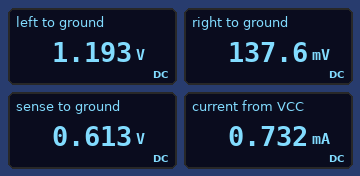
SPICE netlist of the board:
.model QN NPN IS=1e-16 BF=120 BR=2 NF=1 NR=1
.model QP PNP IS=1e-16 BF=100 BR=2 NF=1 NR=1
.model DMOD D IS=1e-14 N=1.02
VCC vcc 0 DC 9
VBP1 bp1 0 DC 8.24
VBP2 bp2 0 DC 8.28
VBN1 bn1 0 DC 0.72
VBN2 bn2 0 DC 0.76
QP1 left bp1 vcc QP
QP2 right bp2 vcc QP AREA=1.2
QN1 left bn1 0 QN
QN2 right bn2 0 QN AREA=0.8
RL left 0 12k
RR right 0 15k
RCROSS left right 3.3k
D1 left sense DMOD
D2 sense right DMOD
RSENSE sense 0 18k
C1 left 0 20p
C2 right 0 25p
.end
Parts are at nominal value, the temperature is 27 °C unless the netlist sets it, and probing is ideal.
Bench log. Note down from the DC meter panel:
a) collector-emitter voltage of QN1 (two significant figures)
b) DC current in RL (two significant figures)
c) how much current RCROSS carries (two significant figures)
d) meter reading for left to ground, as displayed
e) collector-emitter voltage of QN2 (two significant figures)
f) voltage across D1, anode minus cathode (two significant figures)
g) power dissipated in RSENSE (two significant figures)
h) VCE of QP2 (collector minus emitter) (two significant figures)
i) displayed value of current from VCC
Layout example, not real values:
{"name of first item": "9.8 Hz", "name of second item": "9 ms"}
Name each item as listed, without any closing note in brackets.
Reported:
{"collector-emitter voltage of QN1": "1.2 V", "DC current in RL": "99 µA", "how much current RCROSS carries": "320 µA", "meter reading for left to ground, as displayed": "1.193 V", "collector-emitter voltage of QN2": "140 mV", "voltage across D1, anode minus cathode": "580 mV", "power dissipated in RSENSE": "21 µW", "VCE of QP2 (collector minus emitter)": "-8.9 V", "displayed value of current from VCC": "0.732 mA"}
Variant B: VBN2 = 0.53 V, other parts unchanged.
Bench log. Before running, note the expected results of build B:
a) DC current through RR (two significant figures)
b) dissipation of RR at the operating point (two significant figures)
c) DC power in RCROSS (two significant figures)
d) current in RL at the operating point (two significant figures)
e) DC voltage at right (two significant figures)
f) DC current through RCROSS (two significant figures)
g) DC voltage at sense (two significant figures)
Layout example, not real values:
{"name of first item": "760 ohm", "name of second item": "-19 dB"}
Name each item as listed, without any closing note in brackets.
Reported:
{"DC current through RR": "200 µA", "dissipation of RR at the operating point": "590 µW", "DC power in RCROSS": "8.6 µW", "current in RL at the operating point": "260 µA", "DC voltage at right": "3.0 V", "DC current through RCROSS": "51 µA", "DC voltage at sense": "2.5 V"}
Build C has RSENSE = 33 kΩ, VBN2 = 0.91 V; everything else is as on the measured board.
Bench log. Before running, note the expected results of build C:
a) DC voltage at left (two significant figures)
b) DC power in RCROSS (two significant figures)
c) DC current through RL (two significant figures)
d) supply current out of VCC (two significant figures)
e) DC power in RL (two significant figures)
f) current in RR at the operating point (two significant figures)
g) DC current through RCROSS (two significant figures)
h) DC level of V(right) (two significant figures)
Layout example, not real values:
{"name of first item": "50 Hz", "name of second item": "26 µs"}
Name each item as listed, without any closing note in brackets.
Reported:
{"DC voltage at left": "1.1 V", "DC power in RCROSS": "370 µW", "DC current through RL": "93 µA", "supply current out of VCC": "730 µA", "DC power in RL": "100 µW", "current in RR at the operating point": "320 nA", "DC current through RCROSS": "340 µA", "DC level of V(right)": "4.8 mV"}
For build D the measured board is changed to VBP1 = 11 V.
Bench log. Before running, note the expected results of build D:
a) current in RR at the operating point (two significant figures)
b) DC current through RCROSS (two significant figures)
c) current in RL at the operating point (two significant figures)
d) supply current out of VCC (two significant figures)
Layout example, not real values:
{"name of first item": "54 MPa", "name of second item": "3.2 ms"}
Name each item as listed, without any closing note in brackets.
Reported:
{"current in RR at the operating point": "970 nA", "DC current through RCROSS": "1.2 µA", "current in RL at the operating point": "880 nA", "supply current out of VCC": "150 µA"}
